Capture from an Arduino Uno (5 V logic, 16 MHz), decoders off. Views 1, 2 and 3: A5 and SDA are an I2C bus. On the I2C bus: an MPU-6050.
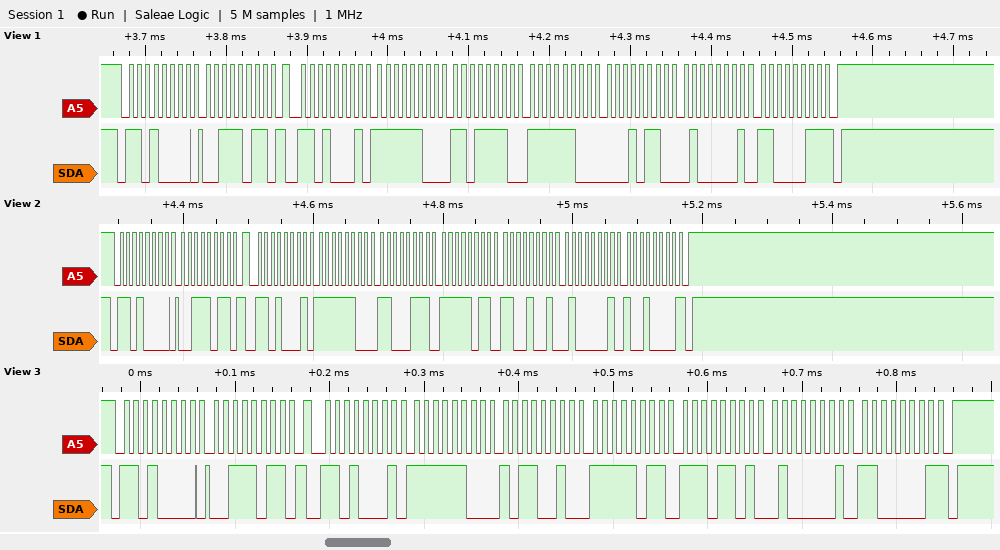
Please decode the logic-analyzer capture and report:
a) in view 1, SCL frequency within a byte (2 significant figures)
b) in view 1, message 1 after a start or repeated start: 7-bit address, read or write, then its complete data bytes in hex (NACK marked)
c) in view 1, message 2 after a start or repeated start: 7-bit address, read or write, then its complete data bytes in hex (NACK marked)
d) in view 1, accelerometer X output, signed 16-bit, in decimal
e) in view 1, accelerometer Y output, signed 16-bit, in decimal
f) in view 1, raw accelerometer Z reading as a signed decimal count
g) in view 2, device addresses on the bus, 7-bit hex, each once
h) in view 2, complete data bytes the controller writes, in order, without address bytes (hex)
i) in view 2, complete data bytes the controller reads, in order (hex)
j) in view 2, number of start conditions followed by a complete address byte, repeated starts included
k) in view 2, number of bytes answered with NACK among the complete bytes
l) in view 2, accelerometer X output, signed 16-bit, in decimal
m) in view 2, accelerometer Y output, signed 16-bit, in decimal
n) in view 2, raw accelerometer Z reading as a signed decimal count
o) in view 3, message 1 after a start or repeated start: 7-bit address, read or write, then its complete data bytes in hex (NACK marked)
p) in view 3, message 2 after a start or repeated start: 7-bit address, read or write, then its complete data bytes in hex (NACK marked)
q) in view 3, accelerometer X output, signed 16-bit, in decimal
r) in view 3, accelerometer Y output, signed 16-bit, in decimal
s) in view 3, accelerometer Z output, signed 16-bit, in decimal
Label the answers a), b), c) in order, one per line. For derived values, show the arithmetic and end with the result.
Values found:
a) 100 kHz
b) 0x68 write: 3B
c) 0x68 read: FC DE FC 16 41 C3 NACK
d) 0xFCDE = -802
e) 0xFC16 = -1002
f) 0x41C3 = 16835
g) 0x68
h) 3B
i) FC C7 FB C9 41 90
j) 2
k) 1
l) 0xFCC7 = -825
m) 0xFBC9 = -1079
n) 0x4190 = 16784
o) 0x68 write: 3B
p) 0x68 read: FC B2 FB ED 41 C1 NACK
q) 0xFCB2 = -846
r) 0xFBED = -1043
s) 0x41C1 = 16833
